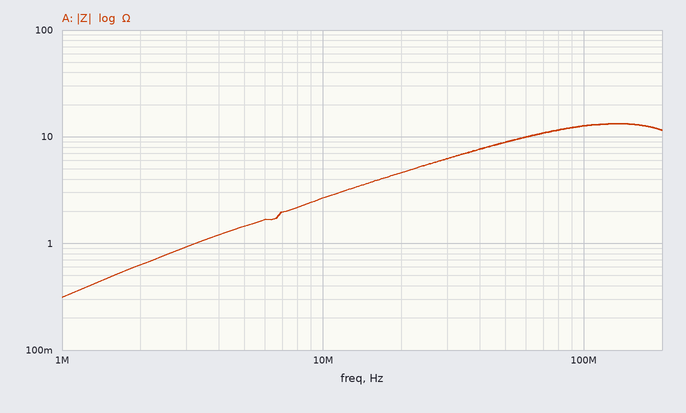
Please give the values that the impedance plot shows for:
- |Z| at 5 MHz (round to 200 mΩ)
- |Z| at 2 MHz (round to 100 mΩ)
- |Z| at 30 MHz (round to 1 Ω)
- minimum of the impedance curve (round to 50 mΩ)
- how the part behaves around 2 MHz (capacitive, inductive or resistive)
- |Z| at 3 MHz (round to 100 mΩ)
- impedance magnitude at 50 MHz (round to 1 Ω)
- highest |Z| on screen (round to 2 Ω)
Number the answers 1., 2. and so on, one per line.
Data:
1. 1.4 Ω
2. 600 mΩ
3. 6 Ω
4. 300 mΩ
5. inductive
6. 900 mΩ
7. 9 Ω
8. 14 Ω
